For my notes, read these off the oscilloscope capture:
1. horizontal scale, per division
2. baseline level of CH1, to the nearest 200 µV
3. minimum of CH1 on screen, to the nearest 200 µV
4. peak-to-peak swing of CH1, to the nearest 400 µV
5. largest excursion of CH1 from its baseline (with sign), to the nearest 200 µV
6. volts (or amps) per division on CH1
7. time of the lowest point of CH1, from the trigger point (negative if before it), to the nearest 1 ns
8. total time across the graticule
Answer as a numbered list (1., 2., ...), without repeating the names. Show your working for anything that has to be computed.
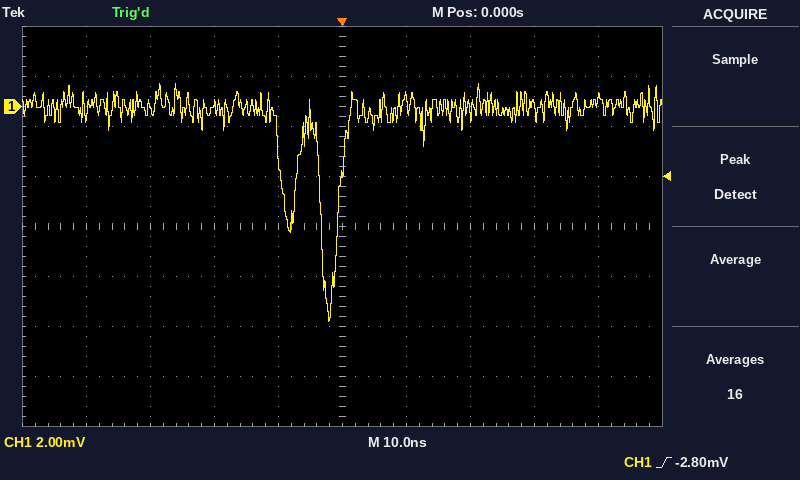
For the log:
1. 10 ns
2. 0.0 mV
3. -8.6 mV
4. 9.6 mV
5. -8.6 mV − (0.0 mV) = -8.6 mV
6. 2 mV
7. -2 ns
8. 100 ns
